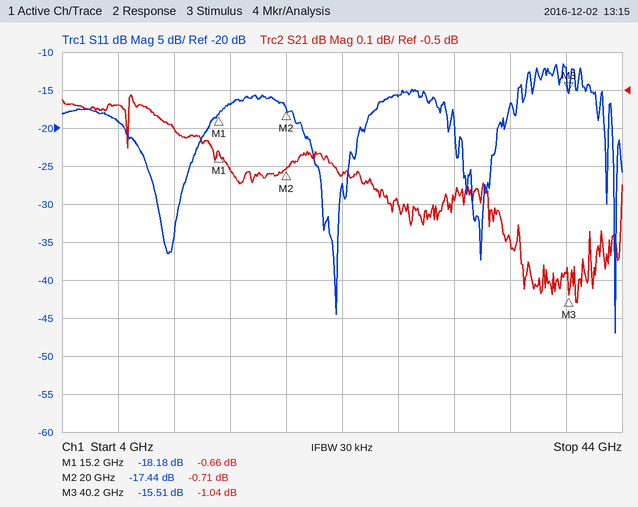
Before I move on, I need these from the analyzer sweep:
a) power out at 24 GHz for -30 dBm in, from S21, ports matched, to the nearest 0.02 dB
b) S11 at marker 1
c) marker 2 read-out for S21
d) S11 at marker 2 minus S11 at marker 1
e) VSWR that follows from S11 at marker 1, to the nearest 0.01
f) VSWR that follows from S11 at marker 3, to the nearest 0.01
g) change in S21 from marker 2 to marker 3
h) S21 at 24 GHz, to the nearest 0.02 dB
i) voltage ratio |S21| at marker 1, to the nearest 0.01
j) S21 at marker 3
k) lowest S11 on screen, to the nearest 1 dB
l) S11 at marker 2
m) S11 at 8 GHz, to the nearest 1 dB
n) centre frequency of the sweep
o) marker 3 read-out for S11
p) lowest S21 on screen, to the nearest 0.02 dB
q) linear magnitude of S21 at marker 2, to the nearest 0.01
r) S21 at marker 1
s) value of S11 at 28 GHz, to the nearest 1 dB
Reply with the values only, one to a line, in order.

-30.72 dBm
-18.18 dB
-0.71 dB
0.74 dB
1.28
1.40
-0.33 dB
-0.72 dB
0.93
-1.04 dB
-47 dB
-17.44 dB
-19 dB
24 GHz
-15.51 dB
-1.06 dB
0.92
-0.66 dB
-16 dB
